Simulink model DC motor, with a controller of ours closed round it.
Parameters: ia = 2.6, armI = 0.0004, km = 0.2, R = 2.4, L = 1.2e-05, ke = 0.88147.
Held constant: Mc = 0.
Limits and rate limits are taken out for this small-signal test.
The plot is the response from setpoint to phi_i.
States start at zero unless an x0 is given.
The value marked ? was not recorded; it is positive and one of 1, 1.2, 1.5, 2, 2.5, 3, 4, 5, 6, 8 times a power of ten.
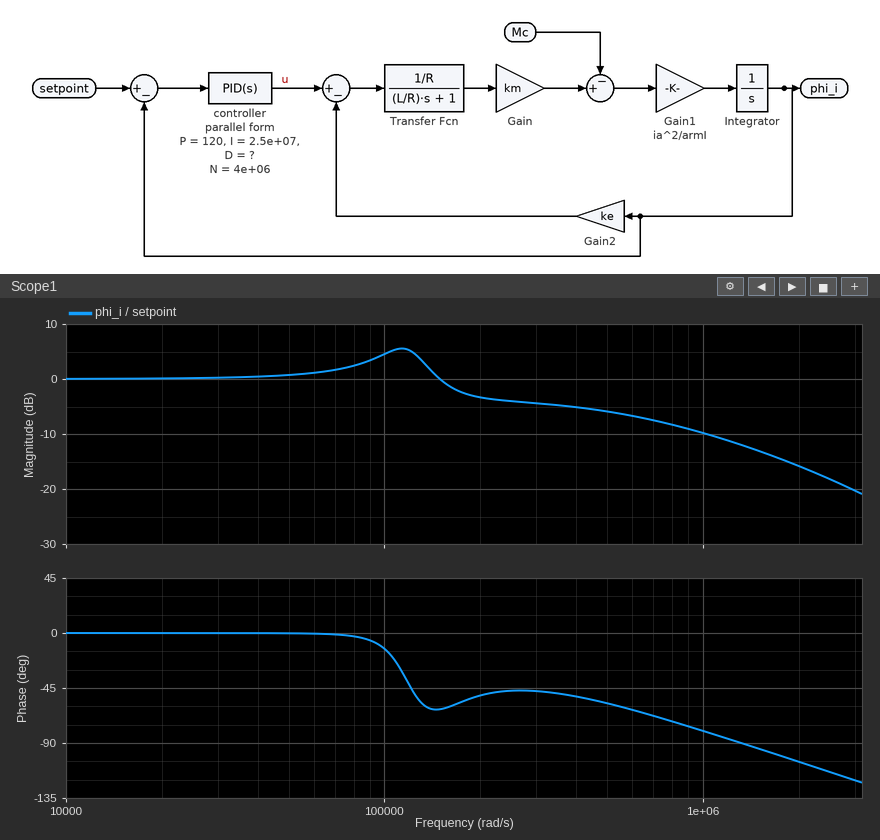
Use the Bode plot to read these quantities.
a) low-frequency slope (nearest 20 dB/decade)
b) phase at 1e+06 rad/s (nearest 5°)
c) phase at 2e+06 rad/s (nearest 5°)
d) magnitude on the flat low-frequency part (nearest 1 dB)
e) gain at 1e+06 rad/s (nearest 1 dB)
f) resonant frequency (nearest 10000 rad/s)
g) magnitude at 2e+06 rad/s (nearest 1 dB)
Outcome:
0 dB/decade
-80°
-105°
0 dB
-10 dB
110000 rad/s
-16 dB
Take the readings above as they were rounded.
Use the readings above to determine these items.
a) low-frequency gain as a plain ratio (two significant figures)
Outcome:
1.0
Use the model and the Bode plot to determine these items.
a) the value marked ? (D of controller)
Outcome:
0.0012
